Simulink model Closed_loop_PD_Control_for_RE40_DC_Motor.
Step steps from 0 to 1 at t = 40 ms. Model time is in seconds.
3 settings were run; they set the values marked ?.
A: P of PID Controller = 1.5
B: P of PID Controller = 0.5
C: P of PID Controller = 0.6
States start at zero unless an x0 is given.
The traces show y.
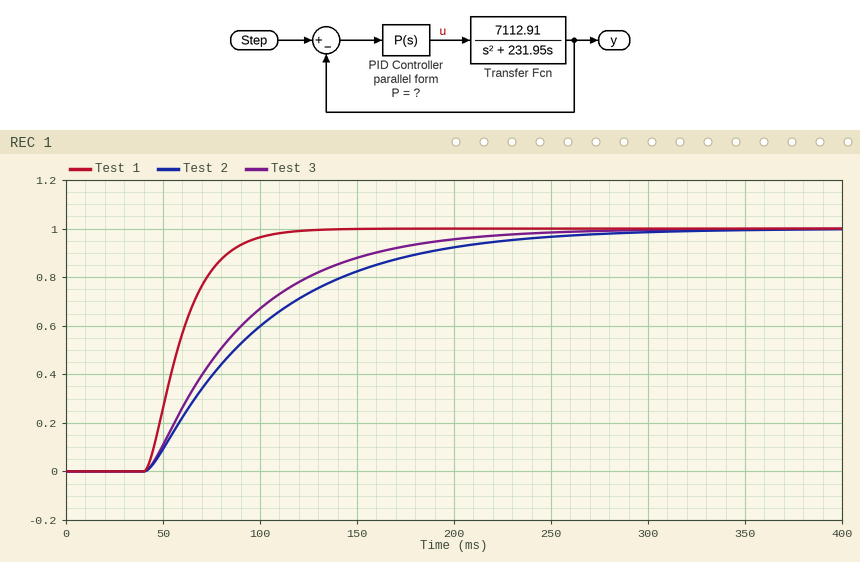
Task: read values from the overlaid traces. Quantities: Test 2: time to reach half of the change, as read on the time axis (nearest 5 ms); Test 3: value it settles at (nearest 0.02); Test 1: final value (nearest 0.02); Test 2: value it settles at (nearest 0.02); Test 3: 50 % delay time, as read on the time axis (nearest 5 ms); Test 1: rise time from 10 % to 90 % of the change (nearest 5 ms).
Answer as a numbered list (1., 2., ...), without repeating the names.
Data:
1. 85 ms
2. 1.00
3. 1.00
4. 1.00
5. 80 ms
6. 40 ms
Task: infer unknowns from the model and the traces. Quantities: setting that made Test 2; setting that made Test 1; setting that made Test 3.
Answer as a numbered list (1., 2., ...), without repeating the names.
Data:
1. B
2. A
3. C
